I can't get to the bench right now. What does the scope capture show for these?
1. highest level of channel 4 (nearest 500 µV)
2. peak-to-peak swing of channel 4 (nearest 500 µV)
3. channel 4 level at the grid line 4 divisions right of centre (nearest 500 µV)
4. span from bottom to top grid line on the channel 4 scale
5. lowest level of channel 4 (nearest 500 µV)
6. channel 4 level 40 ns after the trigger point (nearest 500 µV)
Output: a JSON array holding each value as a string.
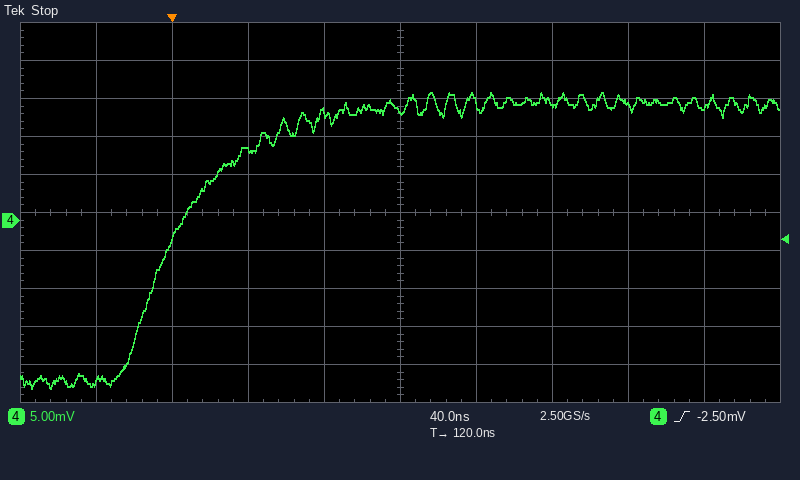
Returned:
["17.0 mV", "39.0 mV", "15.0 mV", "50 mV", "-22.0 mV", "9.0 mV"]
